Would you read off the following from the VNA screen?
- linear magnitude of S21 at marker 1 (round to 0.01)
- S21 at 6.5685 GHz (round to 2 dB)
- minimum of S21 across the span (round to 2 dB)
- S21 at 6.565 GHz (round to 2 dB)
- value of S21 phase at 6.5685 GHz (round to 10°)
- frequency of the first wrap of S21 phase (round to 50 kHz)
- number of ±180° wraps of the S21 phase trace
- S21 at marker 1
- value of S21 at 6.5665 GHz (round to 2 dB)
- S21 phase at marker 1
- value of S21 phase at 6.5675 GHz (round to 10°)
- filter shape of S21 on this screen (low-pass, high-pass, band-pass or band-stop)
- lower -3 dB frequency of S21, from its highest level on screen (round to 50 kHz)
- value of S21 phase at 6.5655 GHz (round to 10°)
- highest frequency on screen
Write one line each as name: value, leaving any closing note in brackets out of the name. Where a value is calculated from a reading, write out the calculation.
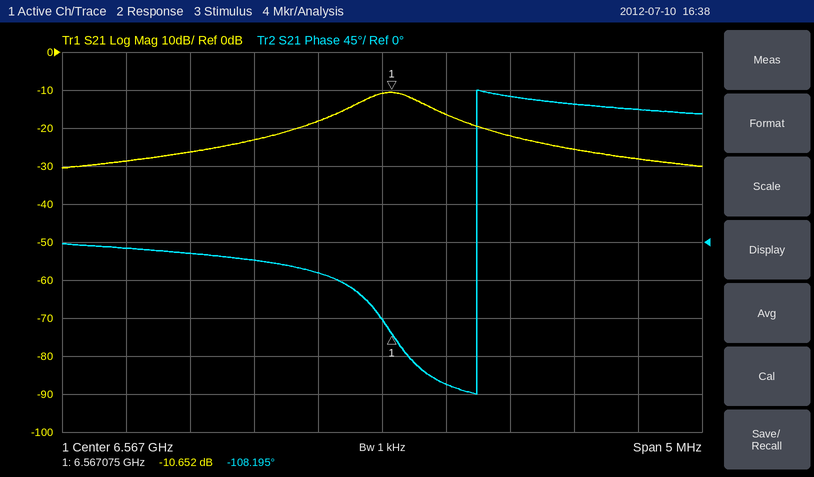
linear magnitude of S21 at marker 1: 10^(-10.652/20) ≈ 0.29
S21 at 6.5685 GHz: -26 dB
minimum of S21 across the span: -30 dB
S21 at 6.565 GHz: -28 dB
value of S21 phase at 6.5685 GHz: 160°
frequency of the first wrap of S21 phase: 6.56775 GHz
number of ±180° wraps of the S21 phase trace: 1
S21 at marker 1: -10.652 dB
value of S21 at 6.5665 GHz: -18 dB
S21 phase at marker 1: -108.195°
value of S21 phase at 6.5675 GHz: -170°
filter shape of S21 on this screen: band-pass
lower -3 dB frequency of S21, from its highest level on screen: 6.56680 GHz
value of S21 phase at 6.5655 GHz: -10°
highest frequency on screen: 6.5695 GHz
